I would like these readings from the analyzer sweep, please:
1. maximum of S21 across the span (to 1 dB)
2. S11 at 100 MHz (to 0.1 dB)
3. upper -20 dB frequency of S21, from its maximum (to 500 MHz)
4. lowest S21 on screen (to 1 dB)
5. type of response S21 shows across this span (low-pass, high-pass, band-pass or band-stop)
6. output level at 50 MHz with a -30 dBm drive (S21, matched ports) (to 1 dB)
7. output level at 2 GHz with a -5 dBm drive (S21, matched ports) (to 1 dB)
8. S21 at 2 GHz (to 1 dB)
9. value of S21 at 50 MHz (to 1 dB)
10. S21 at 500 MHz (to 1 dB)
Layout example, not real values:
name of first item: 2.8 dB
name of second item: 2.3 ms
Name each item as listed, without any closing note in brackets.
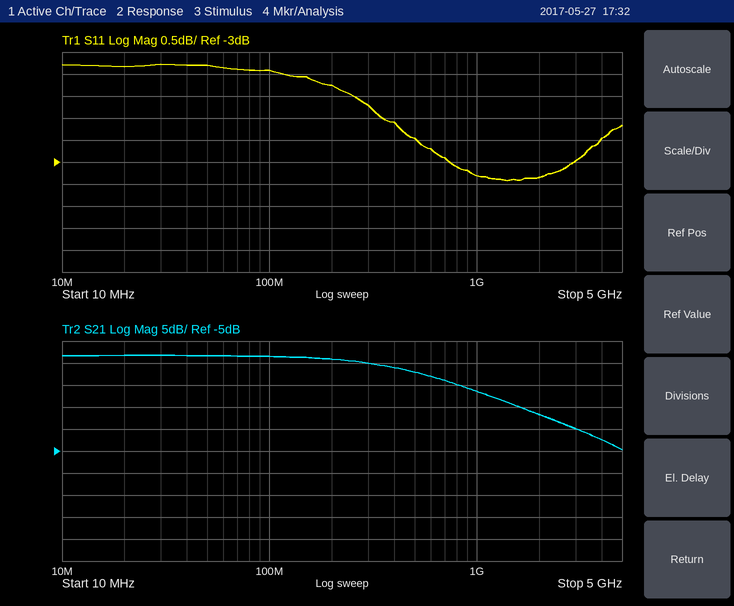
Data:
maximum of S21 across the span: 17 dB
S11 at 100 MHz: -0.9 dB
upper -20 dB frequency of S21, from its maximum: 4.5 GHz
lowest S21 on screen: -5 dB
type of response S21 shows across this span: low-pass
output level at 50 MHz with a -30 dBm drive (S21, matched ports): -13 dBm
output level at 2 GHz with a -5 dBm drive (S21, matched ports): -2 dBm
S21 at 2 GHz: 3 dB
value of S21 at 50 MHz: 17 dB
S21 at 500 MHz: 13 dB
